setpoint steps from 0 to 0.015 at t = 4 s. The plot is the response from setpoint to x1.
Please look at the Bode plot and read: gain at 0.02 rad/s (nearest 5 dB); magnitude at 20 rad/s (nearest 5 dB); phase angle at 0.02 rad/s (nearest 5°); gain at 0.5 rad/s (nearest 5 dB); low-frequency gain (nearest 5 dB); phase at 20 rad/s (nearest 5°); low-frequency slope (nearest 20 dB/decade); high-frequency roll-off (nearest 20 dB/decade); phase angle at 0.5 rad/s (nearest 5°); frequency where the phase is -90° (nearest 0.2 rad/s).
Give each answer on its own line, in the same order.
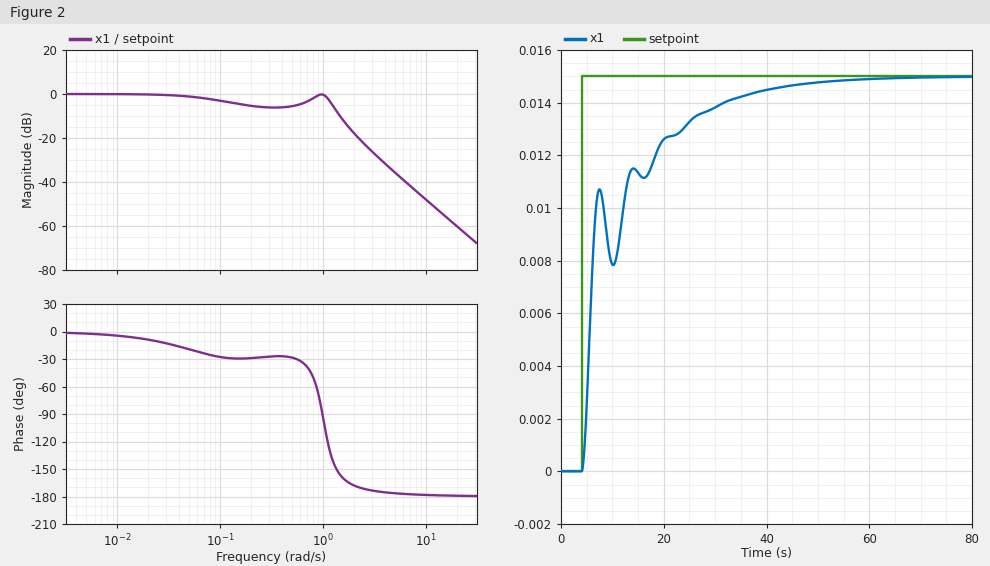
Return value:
0 dB
-60 dB
-10°
-5 dB
0 dB
-180°
0 dB/decade
-40 dB/decade
-30°
1.0 rad/s
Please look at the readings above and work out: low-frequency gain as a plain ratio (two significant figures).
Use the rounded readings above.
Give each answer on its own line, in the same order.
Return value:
1.0
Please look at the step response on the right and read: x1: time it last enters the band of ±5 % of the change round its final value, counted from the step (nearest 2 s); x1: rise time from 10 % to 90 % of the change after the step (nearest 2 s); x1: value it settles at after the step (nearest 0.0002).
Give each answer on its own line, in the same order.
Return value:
32 s
22 s
0.0150
